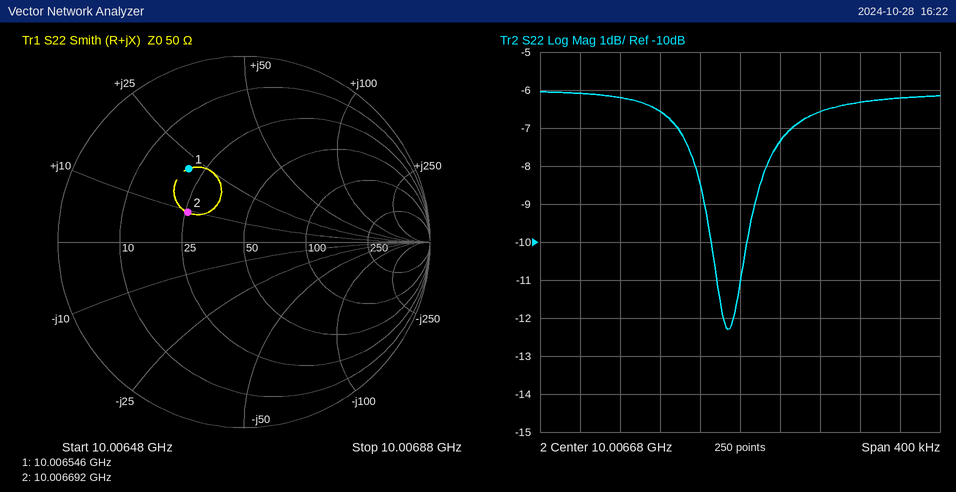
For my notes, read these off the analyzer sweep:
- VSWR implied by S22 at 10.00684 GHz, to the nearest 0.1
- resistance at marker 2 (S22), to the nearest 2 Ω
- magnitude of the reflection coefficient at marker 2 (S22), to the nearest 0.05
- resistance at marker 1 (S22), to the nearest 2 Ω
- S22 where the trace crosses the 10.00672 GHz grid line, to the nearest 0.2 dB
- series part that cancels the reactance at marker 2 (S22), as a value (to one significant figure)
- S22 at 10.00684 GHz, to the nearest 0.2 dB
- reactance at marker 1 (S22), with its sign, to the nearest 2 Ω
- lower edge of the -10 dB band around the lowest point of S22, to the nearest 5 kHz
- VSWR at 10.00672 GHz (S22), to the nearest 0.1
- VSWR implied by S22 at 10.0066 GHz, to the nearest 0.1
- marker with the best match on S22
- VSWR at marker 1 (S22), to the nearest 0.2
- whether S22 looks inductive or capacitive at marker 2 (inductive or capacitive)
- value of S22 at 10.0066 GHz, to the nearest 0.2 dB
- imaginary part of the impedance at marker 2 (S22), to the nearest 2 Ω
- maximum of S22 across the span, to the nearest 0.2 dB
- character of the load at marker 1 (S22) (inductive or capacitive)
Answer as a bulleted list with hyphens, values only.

- 2.9
- 26 Ω
- 0.35
- 20 Ω
- -7.4 dB
- 2 pF
- -6.2 dB
- +22 Ω
- 10.006650 GHz
- 2.5
- 2.8
- marker 2
- 3.0
- inductive
- -6.6 dB
- +10 Ω
- -6.0 dB
- inductive
